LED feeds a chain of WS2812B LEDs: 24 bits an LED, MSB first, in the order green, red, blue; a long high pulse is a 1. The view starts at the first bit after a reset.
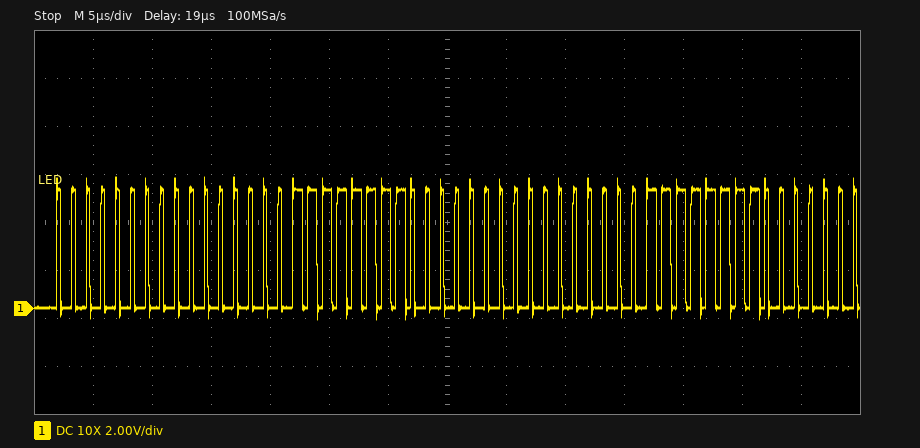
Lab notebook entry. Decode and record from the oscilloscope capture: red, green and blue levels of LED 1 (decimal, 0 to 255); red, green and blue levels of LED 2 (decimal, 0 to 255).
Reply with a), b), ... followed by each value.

a) 0, 0, 255
b) 0, 0, 255
